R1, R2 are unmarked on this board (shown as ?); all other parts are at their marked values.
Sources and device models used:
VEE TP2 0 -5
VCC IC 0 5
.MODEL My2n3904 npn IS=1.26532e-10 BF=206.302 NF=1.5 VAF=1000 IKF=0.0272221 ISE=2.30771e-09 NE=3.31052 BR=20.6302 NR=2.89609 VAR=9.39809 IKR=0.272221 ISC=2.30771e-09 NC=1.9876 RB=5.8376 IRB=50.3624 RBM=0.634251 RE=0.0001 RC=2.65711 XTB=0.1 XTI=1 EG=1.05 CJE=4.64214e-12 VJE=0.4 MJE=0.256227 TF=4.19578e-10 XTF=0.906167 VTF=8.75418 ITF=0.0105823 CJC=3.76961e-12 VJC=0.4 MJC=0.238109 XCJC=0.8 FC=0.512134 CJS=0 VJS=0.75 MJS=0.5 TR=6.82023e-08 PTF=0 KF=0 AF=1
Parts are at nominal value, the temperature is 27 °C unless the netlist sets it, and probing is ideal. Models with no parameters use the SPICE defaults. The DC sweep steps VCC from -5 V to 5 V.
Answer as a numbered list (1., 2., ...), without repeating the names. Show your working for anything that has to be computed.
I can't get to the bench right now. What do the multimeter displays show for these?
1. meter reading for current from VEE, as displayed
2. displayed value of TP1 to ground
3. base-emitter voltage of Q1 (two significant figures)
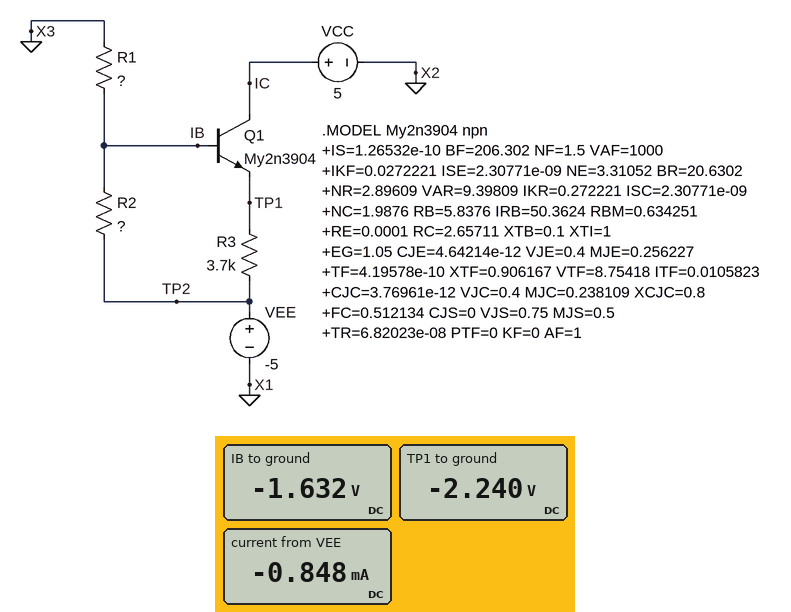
1. -0.848 mA
2. -2.240 V
3. -1.632 V - (-2.24 V) = 610 mV
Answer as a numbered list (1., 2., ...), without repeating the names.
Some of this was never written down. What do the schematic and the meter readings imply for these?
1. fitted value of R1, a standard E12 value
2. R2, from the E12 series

1. 15 kΩ
2. 33 kΩ
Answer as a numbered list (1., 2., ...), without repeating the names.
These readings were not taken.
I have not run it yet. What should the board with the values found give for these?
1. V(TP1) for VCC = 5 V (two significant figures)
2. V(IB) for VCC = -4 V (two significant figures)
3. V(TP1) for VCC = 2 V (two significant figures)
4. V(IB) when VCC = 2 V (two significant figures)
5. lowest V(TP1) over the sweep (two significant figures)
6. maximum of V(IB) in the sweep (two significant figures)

1. -2.2 V
2. -3.4 V
3. -2.2 V
4. -1.6 V
5. -4.9 V
6. -1.6 V
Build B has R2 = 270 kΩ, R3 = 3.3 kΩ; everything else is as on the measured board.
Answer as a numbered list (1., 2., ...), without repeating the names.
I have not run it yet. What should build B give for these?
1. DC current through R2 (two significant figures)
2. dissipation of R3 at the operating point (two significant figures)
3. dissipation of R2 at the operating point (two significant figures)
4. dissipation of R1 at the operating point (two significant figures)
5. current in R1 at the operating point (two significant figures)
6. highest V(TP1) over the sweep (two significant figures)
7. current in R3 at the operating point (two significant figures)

1. 17 µA
2. 4.8 mW
3. 78 µW
4. 11 µW
5. 27 µA
6. -1.0 V
7. 1.2 mA
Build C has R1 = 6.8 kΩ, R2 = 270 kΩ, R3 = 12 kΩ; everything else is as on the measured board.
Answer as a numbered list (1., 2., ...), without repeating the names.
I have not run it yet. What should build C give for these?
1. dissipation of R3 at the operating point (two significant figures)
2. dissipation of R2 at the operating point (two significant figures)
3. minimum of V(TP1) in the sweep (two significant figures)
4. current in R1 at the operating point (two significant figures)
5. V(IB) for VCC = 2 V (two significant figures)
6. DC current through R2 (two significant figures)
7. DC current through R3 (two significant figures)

1. 1.5 mW
2. 87 µW
3. -4.8 V
4. 22 µA
5. -150 mV
6. 18 µA
7. 360 µA
